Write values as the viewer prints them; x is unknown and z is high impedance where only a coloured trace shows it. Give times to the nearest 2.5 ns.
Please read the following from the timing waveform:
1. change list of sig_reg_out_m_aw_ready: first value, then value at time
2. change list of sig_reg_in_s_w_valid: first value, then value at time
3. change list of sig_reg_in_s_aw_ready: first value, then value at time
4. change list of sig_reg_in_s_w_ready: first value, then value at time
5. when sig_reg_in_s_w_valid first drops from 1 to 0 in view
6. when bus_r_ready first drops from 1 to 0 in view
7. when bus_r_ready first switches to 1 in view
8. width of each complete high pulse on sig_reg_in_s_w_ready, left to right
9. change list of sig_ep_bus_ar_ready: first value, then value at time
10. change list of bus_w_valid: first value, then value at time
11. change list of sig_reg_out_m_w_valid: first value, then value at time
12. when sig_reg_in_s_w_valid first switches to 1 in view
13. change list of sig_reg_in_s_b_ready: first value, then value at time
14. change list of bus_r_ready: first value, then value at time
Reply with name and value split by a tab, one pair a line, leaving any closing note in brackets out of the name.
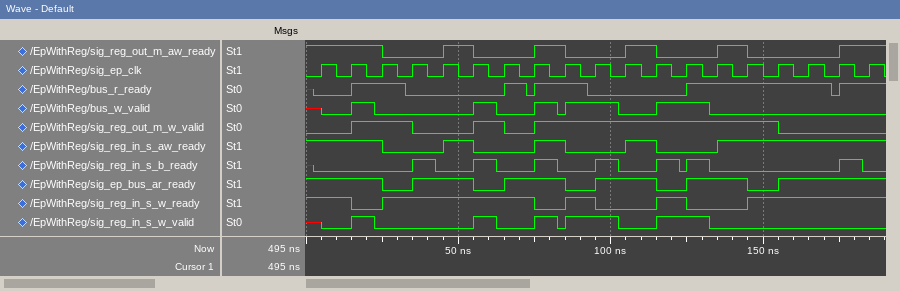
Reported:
change list of sig_reg_out_m_aw_ready: first value, then value at time	1, 0 at 25 ns, 1 at 45 ns, 0 at 55 ns, 1 at 75 ns, 0 at 85 ns, 1 at 105 ns, 0 at 115 ns, 1 at 135 ns, 0 at 145 ns, 1 at 175 ns
change list of sig_reg_in_s_w_valid: first value, then value at time	x, 0 at 5 ns, 1 at 15 ns, 0 at 22.5 ns, 1 at 55 ns, 0 at 62.5 ns, 1 at 75 ns, 0 at 82.5 ns, 1 at 85 ns, 0 at 102.5 ns, 1 at 115 ns, 0 at 132.5 ns
change list of sig_reg_in_s_aw_ready: first value, then value at time	1, 0 at 25 ns, 1 at 45 ns, 0 at 55 ns, 1 at 75 ns, 0 at 85 ns, 1 at 105 ns, 0 at 115 ns, 1 at 135 ns
change list of sig_reg_in_s_w_ready: first value, then value at time	1, 0 at 15 ns, 1 at 25 ns, 0 at 75 ns, 1 at 85 ns, 0 at 95 ns, 1 at 115 ns, 0 at 125 ns, 1 at 145 ns
when sig_reg_in_s_w_valid first drops from 1 to 0 in view	22.5 ns
when bus_r_ready first drops from 1 to 0 in view	32.5 ns
when bus_r_ready first switches to 1 in view	15 ns
width of each complete high pulse on sig_reg_in_s_w_ready, left to right	50 ns, 10 ns, 10 ns
change list of sig_ep_bus_ar_ready: first value, then value at time	1, 0 at 25 ns, 1 at 35 ns, 0 at 55 ns, 1 at 65 ns, 0 at 85 ns, 1 at 95 ns, 0 at 115 ns, 1 at 125 ns, 0 at 145 ns, 1 at 155 ns
change list of bus_w_valid: first value, then value at time	x, 0 at 5 ns, 1 at 15 ns, 0 at 22.5 ns, 1 at 55 ns, 0 at 62.5 ns, 1 at 75 ns, 0 at 82.5 ns, 1 at 85 ns, 0 at 102.5 ns, 1 at 115 ns, 0 at 132.5 ns
change list of sig_reg_out_m_w_valid: first value, then value at time	0, 1 at 15 ns, 0 at 35 ns, 1 at 55 ns, 0 at 65 ns, 1 at 75 ns, 0 at 155 ns
when sig_reg_in_s_w_valid first switches to 1 in view	15 ns
change list of sig_reg_in_s_b_ready: first value, then value at time	x, 0 at 2.5 ns, 1 at 35 ns, 0 at 42.5 ns, 1 at 55 ns, 0 at 62.5 ns, 1 at 75 ns, 0 at 82.5 ns, 1 at 95 ns, 0 at 102.5 ns, 1 at 115 ns, 0 at 122.5 ns, 1 at 125 ns, 0 at 132.5 ns, 1 at 175 ns, 0 at 182.5 ns
change list of bus_r_ready: first value, then value at time	x, 0 at 2.5 ns, 1 at 15 ns, 0 at 32.5 ns, 1 at 65 ns, 0 at 72.5 ns, 1 at 75 ns, 0 at 92.5 ns, 1 at 125 ns, 0 at 172.5 ns, 1 at 175 ns
